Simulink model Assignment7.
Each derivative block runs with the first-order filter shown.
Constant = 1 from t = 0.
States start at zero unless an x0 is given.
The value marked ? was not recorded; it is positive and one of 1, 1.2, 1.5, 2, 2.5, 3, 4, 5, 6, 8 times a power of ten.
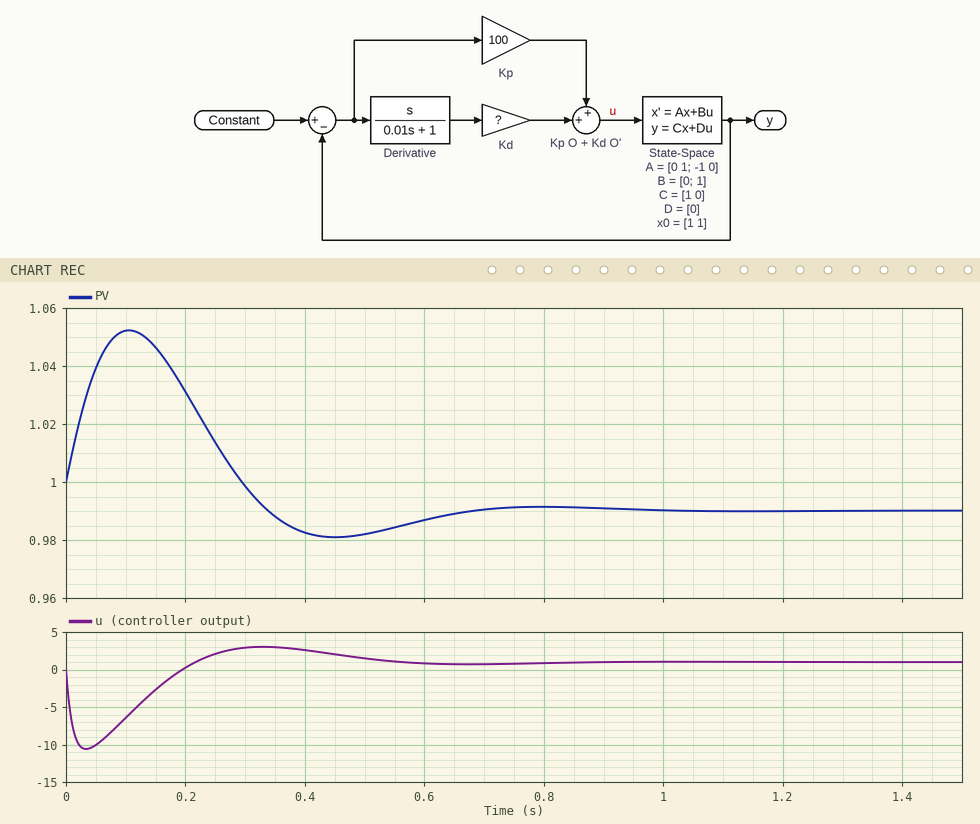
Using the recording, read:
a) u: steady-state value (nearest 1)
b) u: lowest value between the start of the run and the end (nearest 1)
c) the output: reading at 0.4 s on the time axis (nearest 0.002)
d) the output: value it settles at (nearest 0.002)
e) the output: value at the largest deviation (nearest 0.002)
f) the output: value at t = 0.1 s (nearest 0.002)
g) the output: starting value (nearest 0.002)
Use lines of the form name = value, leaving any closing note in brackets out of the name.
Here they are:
u: steady-state value = 1
u: lowest value between the start of the run and the end = -11
the output: reading at 0.4 s on the time axis = 0.982
the output: value it settles at = 0.990
the output: value at the largest deviation = 1.052
the output: value at t = 0.1 s = 1.052
the output: starting value = 1.000
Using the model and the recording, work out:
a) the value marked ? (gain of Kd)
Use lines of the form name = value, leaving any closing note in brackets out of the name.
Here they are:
the value marked ? = 10
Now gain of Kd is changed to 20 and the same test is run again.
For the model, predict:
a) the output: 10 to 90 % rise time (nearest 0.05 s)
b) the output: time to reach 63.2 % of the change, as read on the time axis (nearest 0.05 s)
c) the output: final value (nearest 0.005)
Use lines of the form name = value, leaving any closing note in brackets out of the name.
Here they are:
the output: 10 to 90 % rise time = 0.30 s
the output: time to reach 63.2 % of the change, as read on the time axis = 0.50 s
the output: final value = 0.990
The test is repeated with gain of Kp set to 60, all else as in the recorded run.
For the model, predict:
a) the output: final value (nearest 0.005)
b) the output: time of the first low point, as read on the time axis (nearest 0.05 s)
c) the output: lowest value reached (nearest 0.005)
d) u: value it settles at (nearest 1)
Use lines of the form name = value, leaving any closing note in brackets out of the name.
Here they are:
the output: final value = 0.985
the output: time of the first low point, as read on the time axis = 0.65 s
the output: lowest value reached = 0.980
u: value it settles at = 1
